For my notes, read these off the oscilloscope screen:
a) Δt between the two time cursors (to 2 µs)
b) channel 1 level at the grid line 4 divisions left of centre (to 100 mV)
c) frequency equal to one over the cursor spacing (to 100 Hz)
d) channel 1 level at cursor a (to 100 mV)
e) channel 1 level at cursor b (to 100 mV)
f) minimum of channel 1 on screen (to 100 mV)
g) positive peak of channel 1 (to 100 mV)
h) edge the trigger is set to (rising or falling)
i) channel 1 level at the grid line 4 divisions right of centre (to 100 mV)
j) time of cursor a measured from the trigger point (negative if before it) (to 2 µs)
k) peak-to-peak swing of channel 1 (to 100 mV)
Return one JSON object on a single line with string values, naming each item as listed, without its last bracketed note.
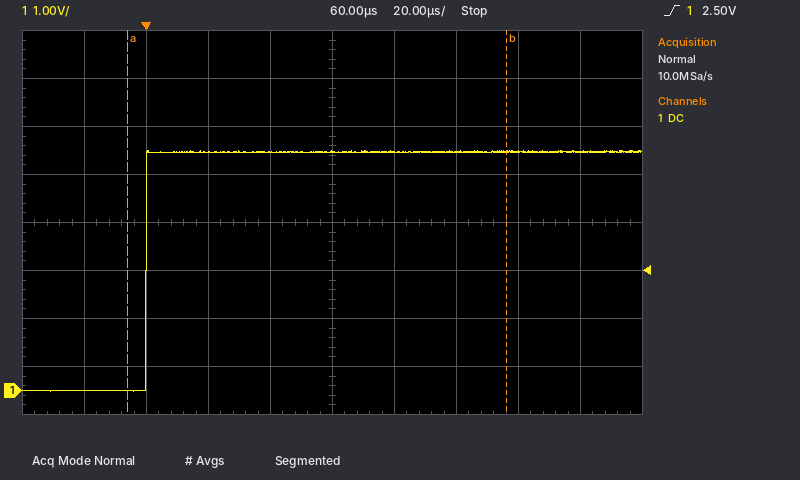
{"Δt between the two time cursors": "122 µs", "channel 1 level at the grid line 4 divisions left of centre": "0.0 V", "frequency equal to one over the cursor spacing": "8.2 kHz", "channel 1 level at cursor a": "0.0 V", "channel 1 level at cursor b": "5.0 V", "minimum of channel 1 on screen": "0.0 V", "positive peak of channel 1": "5.0 V", "edge the trigger is set to": "rising", "channel 1 level at the grid line 4 divisions right of centre": "5.0 V", "time of cursor a measured from the trigger point (negative if before it)": "-6 µs", "peak-to-peak swing of channel 1": "5.0 V"}
